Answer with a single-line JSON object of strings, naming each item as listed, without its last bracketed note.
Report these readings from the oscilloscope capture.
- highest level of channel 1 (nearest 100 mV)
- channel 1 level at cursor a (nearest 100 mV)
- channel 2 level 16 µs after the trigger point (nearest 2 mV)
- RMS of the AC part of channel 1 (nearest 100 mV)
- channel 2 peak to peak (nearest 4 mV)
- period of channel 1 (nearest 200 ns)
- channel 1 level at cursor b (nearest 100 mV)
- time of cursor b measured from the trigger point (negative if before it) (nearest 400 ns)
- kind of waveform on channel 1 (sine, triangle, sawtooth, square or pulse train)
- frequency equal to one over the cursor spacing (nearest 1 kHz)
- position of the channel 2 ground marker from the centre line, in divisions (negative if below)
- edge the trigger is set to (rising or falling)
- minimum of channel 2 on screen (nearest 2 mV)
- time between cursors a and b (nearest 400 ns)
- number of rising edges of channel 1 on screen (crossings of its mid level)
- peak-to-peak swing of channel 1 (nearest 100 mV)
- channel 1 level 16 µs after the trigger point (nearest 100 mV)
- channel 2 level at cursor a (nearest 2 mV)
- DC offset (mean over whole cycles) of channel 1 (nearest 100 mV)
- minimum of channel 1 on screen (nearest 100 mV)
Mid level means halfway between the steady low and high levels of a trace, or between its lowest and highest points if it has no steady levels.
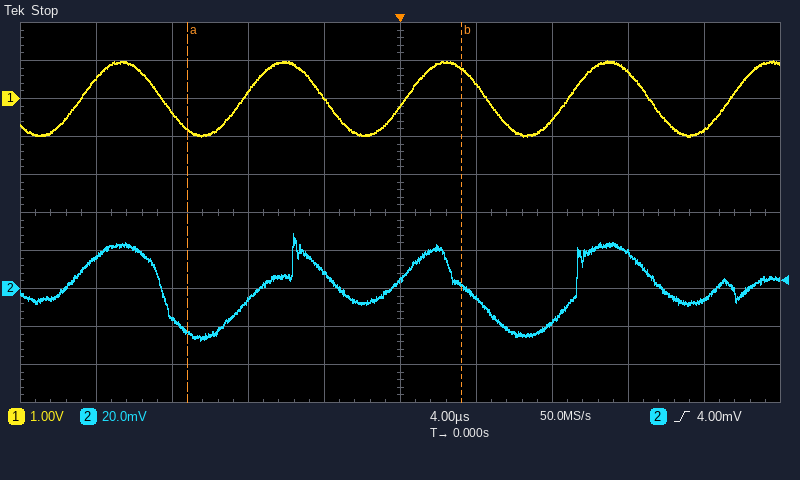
{"highest level of channel 1": "1.0 V", "channel 1 level at cursor a": "-800 mV", "channel 2 level 16 µs after the trigger point": "-6 mV", "RMS of the AC part of channel 1": "700 mV", "channel 2 peak to peak": "56 mV", "period of channel 1": "8.6 µs", "channel 1 level at cursor b": "800 mV", "time of cursor b measured from the trigger point (negative if before it)": "+3.2 µs", "kind of waveform on channel 1": "sine", "frequency equal to one over the cursor spacing": "69 kHz", "position of the channel 2 ground marker from the centre line, in divisions": "-2.0 div", "edge the trigger is set to": "rising", "minimum of channel 2 on screen": "-28 mV", "time between cursors a and b": "14.4 µs", "number of rising edges of channel 1 on screen": "5", "peak-to-peak swing of channel 1": "2.0 V", "channel 1 level 16 µs after the trigger point": "-800 mV", "channel 2 level at cursor a": "-22 mV", "DC offset (mean over whole cycles) of channel 1": "0.0 V", "minimum of channel 1 on screen": "-1.0 V"}
